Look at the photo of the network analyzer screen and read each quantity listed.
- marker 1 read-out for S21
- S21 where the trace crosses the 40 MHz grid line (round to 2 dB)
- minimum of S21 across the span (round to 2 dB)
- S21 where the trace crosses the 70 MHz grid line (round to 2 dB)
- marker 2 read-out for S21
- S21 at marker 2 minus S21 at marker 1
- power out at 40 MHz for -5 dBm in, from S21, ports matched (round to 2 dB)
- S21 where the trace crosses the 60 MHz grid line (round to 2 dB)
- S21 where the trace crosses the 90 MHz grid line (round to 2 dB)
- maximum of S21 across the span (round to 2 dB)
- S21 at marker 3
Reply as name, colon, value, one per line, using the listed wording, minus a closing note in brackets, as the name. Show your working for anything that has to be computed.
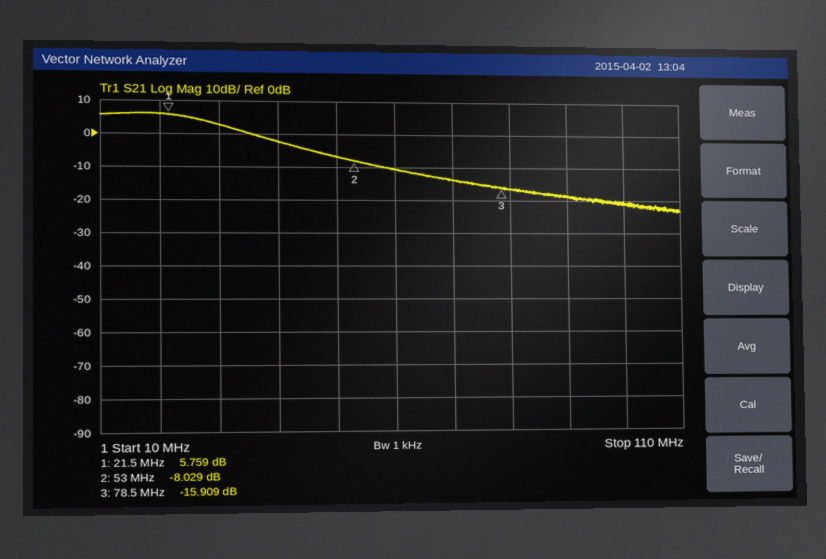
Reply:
marker 1 read-out for S21: 5.759 dB
S21 where the trace crosses the 40 MHz grid line: -2 dB
minimum of S21 across the span: -24 dB
S21 where the trace crosses the 70 MHz grid line: -14 dB
marker 2 read-out for S21: -8.029 dB
S21 at marker 2 minus S21 at marker 1: -8.029 − (5.759) = -13.788 dB
power out at 40 MHz for -5 dBm in, from S21, ports matched: -5 dBm + (-2 dB) = -8 dBm
S21 where the trace crosses the 60 MHz grid line: -10 dB
S21 where the trace crosses the 90 MHz grid line: -18 dB
maximum of S21 across the span: 6 dB
S21 at marker 3: -15.909 dB
